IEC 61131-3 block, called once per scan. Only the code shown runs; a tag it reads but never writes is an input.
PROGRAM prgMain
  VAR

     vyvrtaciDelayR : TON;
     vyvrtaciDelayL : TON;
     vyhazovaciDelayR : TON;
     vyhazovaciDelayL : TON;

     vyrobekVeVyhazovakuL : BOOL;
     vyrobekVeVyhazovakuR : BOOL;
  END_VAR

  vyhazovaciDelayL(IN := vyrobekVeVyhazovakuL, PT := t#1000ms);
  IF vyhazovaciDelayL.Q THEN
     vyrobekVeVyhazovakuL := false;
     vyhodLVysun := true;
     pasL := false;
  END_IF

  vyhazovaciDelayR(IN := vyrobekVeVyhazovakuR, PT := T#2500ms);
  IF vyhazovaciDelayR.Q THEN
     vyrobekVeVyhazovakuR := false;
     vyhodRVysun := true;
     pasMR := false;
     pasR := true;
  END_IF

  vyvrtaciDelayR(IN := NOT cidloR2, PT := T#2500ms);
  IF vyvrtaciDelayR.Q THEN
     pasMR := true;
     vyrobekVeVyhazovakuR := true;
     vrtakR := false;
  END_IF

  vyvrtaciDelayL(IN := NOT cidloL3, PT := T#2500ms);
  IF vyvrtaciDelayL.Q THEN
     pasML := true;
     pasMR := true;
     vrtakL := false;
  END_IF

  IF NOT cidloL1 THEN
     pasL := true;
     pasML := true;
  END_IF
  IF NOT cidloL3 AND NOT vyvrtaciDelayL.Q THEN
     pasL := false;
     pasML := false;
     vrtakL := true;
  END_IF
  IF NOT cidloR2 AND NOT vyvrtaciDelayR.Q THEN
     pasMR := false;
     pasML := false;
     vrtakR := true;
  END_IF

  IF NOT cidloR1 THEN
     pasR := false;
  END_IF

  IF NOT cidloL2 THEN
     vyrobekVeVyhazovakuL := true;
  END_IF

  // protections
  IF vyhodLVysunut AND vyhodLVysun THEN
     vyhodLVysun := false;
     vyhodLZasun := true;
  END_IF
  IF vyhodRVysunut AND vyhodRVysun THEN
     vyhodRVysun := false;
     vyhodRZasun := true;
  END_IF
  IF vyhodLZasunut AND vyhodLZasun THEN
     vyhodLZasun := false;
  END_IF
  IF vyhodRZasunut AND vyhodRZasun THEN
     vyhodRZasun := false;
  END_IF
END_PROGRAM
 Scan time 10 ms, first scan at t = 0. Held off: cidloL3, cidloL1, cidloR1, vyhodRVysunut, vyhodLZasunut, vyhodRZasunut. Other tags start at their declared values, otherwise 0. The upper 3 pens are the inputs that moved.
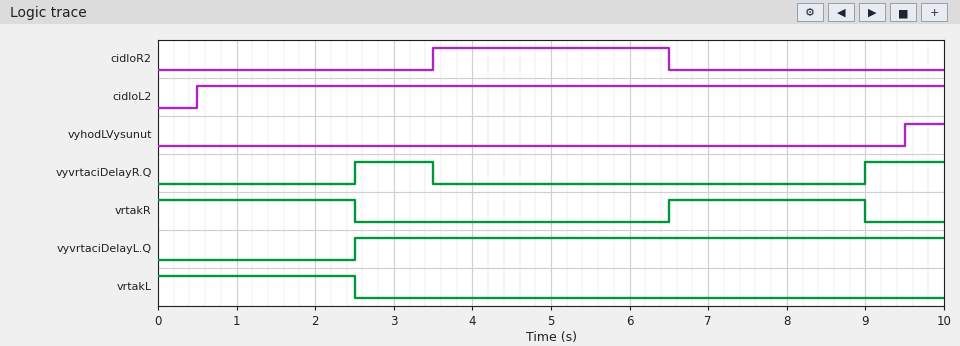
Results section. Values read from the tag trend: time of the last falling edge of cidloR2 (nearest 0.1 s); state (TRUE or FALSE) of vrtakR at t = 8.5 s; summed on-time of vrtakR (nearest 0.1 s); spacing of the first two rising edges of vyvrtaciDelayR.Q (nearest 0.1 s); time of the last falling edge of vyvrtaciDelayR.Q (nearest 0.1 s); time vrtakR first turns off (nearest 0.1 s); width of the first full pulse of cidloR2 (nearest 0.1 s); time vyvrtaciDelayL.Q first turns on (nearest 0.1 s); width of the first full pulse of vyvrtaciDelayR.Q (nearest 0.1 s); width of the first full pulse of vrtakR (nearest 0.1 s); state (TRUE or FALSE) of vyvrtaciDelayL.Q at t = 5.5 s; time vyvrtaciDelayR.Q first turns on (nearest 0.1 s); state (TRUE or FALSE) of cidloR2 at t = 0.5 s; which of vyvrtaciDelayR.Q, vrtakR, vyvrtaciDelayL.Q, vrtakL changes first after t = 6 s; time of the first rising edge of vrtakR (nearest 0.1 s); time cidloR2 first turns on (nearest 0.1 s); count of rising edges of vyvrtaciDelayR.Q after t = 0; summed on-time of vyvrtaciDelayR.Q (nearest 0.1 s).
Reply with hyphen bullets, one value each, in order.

- 6.5 s
- TRUE
- 5.0 s
- 6.5 s
- 3.5 s
- 2.5 s
- 3.0 s
- 2.5 s
- 1.0 s
- 2.5 s
- TRUE
- 2.5 s
- FALSE
- vrtakR
- 6.5 s
- 3.5 s
- 2
- 2.0 s
